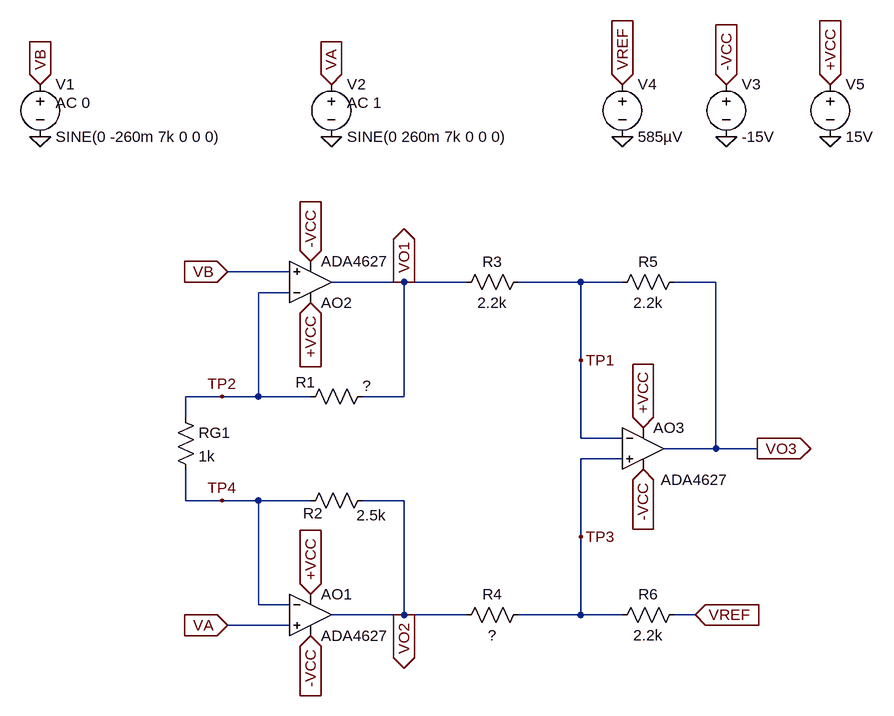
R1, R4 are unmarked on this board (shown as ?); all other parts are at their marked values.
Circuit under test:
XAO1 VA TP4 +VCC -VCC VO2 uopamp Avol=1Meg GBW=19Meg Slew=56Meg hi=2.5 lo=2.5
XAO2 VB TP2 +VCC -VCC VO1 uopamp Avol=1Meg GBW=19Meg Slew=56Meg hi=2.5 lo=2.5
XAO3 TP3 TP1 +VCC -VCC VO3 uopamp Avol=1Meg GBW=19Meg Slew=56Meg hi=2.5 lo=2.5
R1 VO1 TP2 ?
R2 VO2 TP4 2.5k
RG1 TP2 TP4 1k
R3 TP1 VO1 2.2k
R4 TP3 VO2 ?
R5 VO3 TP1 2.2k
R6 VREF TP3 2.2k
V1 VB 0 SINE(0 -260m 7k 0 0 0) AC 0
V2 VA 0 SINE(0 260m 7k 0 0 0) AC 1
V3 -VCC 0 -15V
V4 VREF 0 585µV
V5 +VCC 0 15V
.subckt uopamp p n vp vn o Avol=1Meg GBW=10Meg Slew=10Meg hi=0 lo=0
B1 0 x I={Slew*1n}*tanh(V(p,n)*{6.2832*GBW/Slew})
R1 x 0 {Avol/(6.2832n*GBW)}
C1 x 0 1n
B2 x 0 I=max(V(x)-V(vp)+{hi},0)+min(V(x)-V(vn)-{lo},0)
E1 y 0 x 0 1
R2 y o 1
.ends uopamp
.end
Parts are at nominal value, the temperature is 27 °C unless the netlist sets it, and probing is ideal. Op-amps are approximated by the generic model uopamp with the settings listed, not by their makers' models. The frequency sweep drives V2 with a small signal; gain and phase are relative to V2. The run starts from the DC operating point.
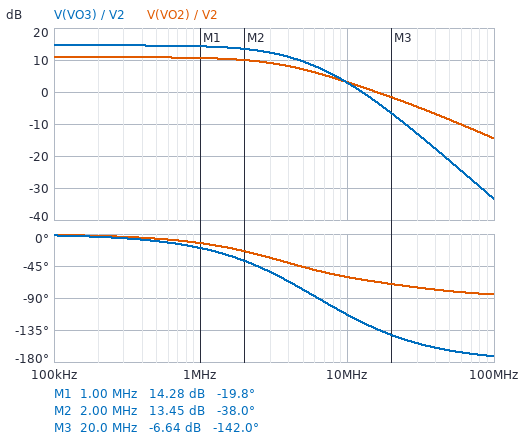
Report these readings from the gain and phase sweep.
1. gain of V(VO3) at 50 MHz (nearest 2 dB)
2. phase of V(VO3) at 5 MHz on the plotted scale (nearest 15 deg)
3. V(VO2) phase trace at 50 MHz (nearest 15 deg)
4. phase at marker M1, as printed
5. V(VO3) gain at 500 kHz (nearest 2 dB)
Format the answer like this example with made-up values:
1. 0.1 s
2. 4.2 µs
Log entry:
1. -22 dB
2. -75 deg
3. -75 deg
4. -19.8 deg
5. 14 dB
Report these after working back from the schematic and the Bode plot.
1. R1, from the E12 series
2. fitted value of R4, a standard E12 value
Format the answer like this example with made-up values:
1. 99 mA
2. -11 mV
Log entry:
1. 1.2 kΩ
2. 1.5 kΩ
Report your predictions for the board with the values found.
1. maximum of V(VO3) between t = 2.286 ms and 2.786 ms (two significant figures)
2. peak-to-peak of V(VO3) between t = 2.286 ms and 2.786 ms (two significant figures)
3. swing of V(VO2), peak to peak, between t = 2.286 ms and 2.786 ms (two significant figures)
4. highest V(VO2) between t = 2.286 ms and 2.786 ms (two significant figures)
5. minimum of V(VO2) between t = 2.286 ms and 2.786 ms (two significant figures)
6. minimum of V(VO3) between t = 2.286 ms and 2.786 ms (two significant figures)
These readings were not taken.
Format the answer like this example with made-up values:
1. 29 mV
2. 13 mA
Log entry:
1. 2.7 V
2. 5.5 V
3. 3.1 V
4. 1.6 V
5. -1.6 V
6. -2.7 V
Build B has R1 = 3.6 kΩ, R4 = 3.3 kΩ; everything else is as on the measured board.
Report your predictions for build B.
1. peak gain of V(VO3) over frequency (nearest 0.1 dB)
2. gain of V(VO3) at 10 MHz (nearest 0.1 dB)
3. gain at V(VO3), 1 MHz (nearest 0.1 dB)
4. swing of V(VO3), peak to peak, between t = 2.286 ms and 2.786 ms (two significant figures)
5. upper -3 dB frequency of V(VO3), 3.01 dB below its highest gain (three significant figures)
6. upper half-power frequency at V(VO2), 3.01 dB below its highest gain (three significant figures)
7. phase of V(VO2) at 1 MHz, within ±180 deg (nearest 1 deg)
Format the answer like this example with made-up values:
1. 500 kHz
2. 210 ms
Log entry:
1. 16.1 dB
2. 0.9 dB
3. 15.5 dB
4. 6.8 V
5. 2.49 MHz
6. 2.85 MHz
7. -17 deg
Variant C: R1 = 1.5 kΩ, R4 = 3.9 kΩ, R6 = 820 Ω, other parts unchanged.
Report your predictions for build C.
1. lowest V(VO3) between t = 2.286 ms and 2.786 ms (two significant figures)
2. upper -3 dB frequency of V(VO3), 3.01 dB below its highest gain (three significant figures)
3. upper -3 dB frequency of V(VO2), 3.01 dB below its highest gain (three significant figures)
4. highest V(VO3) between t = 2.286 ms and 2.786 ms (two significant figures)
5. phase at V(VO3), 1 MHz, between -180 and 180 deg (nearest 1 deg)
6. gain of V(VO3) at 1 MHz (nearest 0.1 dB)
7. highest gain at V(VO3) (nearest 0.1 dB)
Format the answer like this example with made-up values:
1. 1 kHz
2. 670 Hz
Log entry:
1. -1.6 V
2. 3.30 MHz
3. 3.96 MHz
4. 1.6 V
5. -22 deg
6. 8.3 dB
7. 8.7 dB
